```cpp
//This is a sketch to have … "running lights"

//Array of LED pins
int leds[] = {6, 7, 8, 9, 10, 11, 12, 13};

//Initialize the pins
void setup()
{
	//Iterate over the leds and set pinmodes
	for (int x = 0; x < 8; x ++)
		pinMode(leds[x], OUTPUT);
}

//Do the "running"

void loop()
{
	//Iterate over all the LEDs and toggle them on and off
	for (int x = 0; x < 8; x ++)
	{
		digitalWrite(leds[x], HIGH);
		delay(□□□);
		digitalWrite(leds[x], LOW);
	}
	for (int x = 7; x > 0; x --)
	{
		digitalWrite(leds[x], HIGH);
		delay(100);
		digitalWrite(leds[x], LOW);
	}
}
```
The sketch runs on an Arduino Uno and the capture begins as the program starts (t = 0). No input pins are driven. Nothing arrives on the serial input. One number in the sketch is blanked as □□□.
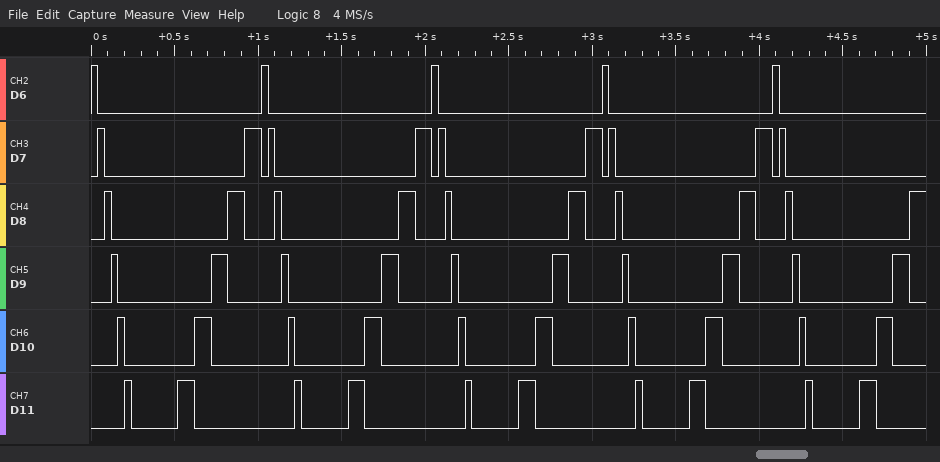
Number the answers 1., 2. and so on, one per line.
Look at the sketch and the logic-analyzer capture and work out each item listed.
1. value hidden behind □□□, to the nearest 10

1. 40
